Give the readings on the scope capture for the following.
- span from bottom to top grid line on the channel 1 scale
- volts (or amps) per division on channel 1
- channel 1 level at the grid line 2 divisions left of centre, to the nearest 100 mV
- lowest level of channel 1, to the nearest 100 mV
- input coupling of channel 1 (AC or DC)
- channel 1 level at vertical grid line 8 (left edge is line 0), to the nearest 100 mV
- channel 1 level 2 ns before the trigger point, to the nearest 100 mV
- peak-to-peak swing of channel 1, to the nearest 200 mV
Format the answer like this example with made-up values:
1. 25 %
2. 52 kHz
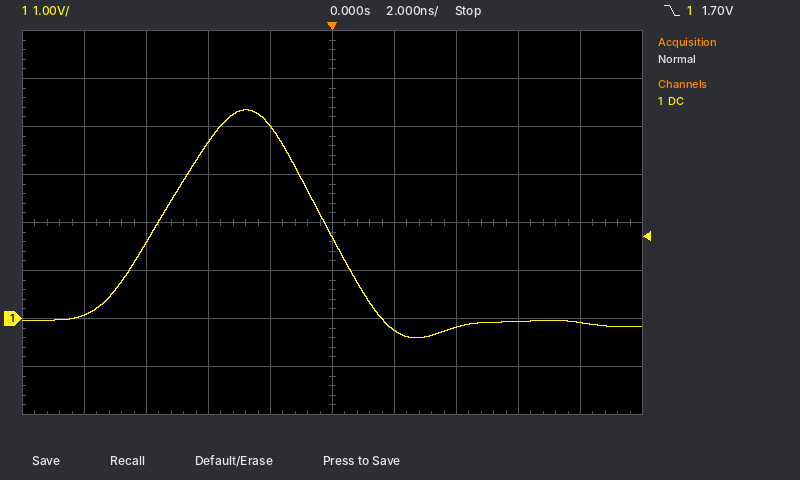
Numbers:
1. 8 V
2. 1 V
3. 3.7 V
4. -400 mV
5. DC
6. -100 mV
7. 4.0 V
8. 4.8 V
